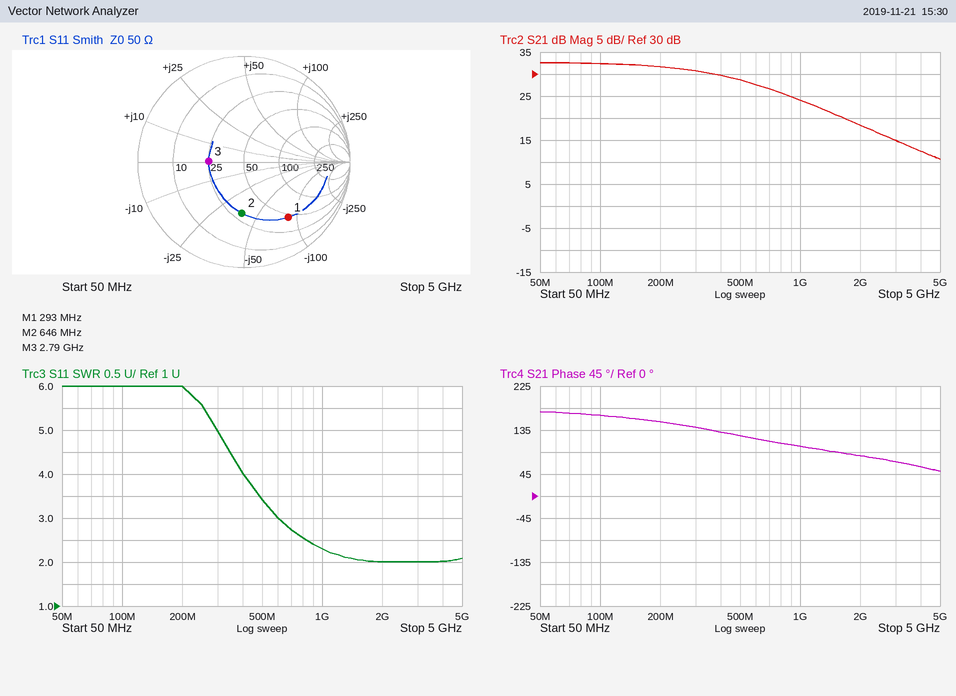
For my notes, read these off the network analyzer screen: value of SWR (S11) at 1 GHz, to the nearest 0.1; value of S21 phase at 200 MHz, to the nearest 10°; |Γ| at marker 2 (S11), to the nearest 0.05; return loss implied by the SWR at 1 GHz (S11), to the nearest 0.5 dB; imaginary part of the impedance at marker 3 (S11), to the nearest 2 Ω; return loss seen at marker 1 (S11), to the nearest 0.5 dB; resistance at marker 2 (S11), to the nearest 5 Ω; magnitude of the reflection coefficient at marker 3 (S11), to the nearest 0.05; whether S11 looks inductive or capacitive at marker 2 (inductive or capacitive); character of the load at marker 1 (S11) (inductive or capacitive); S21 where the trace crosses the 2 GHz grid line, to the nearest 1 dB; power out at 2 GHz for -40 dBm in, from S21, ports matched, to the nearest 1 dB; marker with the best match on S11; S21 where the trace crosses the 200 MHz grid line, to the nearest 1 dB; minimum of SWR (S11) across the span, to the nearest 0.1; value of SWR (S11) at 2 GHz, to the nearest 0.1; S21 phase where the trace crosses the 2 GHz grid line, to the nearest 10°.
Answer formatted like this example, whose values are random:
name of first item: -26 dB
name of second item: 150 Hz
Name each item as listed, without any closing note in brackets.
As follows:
value of SWR (S11) at 1 GHz, to the nearest 0.1: 2.3
value of S21 phase at 200 MHz, to the nearest 10°: 150°
|Γ| at marker 2 (S11), to the nearest 0.05: 0.50
return loss implied by the SWR at 1 GHz (S11), to the nearest 0.5 dB: 8.0 dB
imaginary part of the impedance at marker 3 (S11), to the nearest 2 Ω: 0 Ω
return loss seen at marker 1 (S11), to the nearest 0.5 dB: 3.5 dB
resistance at marker 2 (S11), to the nearest 5 Ω: 30 Ω
magnitude of the reflection coefficient at marker 3 (S11), to the nearest 0.05: 0.35
whether S11 looks inductive or capacitive at marker 2: capacitive
character of the load at marker 1 (S11): capacitive
S21 where the trace crosses the 2 GHz grid line, to the nearest 1 dB: 18 dB
power out at 2 GHz for -40 dBm in, from S21, ports matched, to the nearest 1 dB: -22 dBm
marker with the best match on S11: marker 3
S21 where the trace crosses the 200 MHz grid line, to the nearest 1 dB: 32 dB
minimum of SWR (S11) across the span, to the nearest 0.1: 2.0
value of SWR (S11) at 2 GHz, to the nearest 0.1: 2.0
S21 phase where the trace crosses the 2 GHz grid line, to the nearest 10°: 80°
